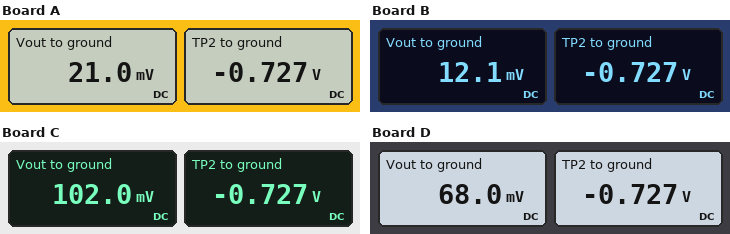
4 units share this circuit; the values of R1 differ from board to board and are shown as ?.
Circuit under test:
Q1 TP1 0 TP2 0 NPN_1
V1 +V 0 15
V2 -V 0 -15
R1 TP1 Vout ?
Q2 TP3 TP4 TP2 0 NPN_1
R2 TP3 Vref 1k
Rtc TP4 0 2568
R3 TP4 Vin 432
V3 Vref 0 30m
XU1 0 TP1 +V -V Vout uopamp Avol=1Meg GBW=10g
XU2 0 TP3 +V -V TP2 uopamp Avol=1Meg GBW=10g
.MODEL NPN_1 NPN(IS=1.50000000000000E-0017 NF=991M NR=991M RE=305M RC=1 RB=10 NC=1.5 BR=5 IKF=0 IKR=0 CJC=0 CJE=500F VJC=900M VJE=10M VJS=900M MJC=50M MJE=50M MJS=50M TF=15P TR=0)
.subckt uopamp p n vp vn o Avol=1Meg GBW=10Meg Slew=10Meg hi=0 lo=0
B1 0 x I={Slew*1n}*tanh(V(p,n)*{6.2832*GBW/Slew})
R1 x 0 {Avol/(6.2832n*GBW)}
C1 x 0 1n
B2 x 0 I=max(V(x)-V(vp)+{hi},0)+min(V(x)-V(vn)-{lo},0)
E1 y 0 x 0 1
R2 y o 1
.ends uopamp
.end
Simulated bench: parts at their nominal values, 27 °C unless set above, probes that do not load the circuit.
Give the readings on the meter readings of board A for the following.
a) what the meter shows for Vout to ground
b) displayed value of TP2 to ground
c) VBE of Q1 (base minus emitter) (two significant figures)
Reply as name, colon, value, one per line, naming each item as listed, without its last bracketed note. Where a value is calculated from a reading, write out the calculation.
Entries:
what the meter shows for Vout to ground: 21.0 mV
displayed value of TP2 to ground: -0.727 V
VBE of Q1 (base minus emitter): 0 V - (-727 mV) = 730 mV
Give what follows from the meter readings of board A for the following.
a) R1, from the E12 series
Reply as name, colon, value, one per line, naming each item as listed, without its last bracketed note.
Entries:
R1, from the E12 series: 680 Ω
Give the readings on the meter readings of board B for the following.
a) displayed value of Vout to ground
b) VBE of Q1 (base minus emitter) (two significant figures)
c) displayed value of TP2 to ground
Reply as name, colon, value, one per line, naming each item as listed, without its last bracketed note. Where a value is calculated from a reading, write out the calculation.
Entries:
displayed value of Vout to ground: 12.1 mV
VBE of Q1 (base minus emitter): 0 V - (-727 mV) = 730 mV
displayed value of TP2 to ground: -0.727 V
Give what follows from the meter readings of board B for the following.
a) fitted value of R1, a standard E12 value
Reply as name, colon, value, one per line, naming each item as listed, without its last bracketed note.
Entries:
fitted value of R1, a standard E12 value: 390 Ω
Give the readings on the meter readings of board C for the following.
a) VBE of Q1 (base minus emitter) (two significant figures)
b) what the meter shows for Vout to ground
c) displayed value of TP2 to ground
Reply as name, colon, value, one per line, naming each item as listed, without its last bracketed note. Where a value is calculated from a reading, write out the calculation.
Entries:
VBE of Q1 (base minus emitter): 0 V - (-727 mV) = 730 mV
what the meter shows for Vout to ground: 102.0 mV
displayed value of TP2 to ground: -0.727 V
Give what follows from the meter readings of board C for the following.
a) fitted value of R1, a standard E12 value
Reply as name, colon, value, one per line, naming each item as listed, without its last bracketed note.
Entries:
fitted value of R1, a standard E12 value: 3.3 kΩ
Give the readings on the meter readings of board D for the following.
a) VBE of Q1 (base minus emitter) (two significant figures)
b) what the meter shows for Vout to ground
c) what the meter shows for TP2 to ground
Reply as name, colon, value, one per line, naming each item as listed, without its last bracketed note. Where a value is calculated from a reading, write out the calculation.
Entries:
VBE of Q1 (base minus emitter): 0 V - (-727 mV) = 730 mV
what the meter shows for Vout to ground: 68.0 mV
what the meter shows for TP2 to ground: -0.727 V
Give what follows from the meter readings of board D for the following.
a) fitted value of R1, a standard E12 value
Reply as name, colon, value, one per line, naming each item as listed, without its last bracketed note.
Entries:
fitted value of R1, a standard E12 value: 2.2 kΩ
